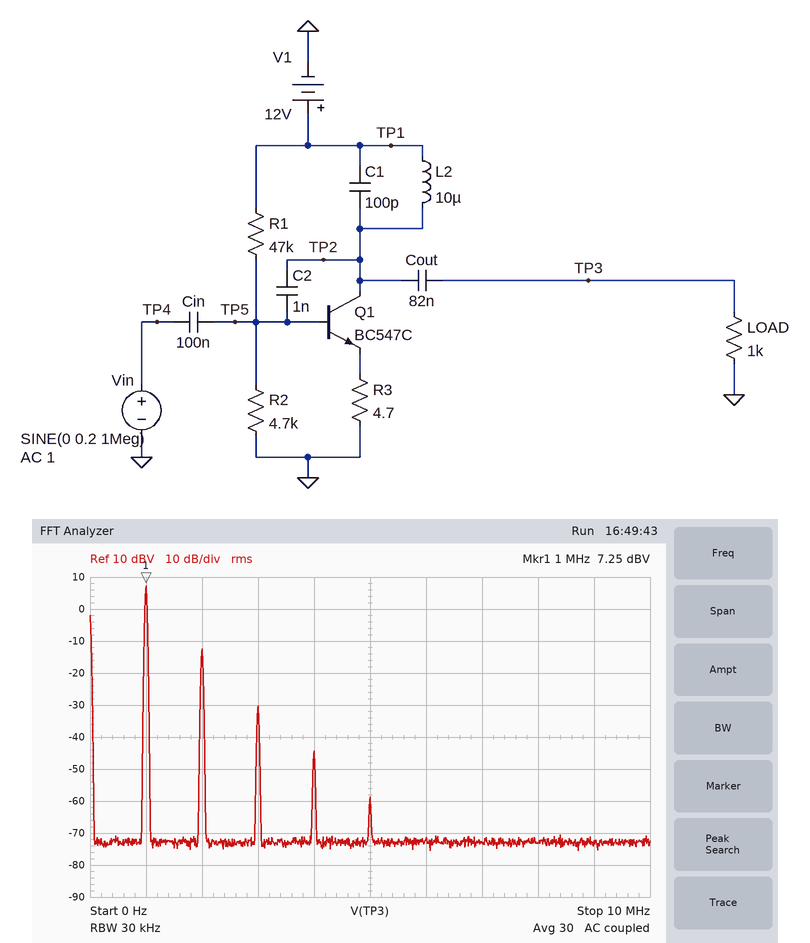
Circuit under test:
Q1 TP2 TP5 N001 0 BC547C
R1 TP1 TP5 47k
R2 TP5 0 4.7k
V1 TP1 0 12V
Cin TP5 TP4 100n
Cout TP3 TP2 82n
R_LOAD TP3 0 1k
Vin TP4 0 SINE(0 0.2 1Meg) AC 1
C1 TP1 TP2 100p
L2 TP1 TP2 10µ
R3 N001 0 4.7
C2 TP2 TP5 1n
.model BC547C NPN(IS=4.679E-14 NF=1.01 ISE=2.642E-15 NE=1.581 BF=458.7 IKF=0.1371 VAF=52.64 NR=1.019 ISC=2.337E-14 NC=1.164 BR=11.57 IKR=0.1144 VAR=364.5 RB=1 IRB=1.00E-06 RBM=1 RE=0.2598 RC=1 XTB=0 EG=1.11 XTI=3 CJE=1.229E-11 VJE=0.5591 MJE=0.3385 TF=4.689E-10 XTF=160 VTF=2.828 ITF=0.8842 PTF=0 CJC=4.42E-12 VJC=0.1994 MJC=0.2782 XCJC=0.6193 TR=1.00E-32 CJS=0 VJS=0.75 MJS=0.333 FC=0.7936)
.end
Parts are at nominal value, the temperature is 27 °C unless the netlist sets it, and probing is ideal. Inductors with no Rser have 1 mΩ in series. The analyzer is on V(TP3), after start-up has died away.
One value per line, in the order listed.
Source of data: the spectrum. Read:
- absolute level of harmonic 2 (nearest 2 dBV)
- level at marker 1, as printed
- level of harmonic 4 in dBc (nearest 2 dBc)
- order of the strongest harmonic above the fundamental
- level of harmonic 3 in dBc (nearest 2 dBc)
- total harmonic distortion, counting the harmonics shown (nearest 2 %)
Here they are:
-12 dBV
7.25 dBV
-52 dBc
2
-38 dBc
10 %
